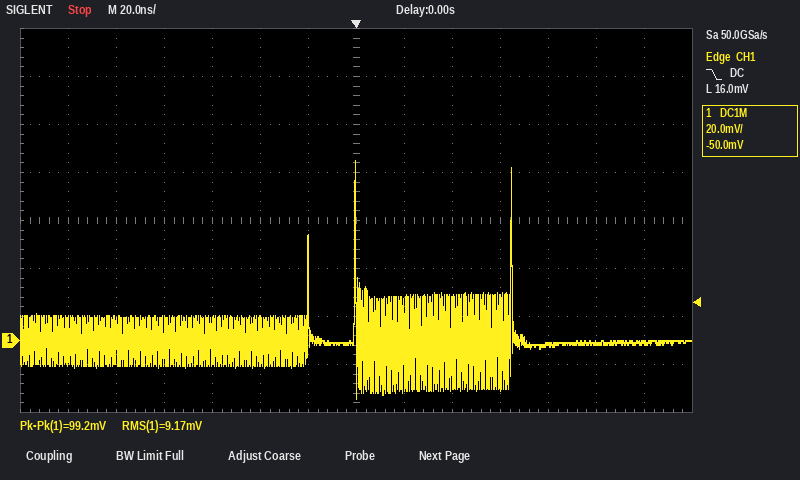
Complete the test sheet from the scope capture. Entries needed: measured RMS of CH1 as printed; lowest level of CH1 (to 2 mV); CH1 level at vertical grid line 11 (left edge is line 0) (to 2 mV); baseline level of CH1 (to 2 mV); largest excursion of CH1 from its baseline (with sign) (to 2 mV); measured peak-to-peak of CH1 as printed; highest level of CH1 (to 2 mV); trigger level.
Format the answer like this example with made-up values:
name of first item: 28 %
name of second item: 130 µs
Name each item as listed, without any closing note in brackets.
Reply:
measured RMS of CH1 as printed: 9.17 mV
lowest level of CH1: -24 mV
CH1 level at vertical grid line 11 (left edge is line 0): -2 mV
baseline level of CH1: 0 mV
largest excursion of CH1 from its baseline (with sign): +76 mV
measured peak-to-peak of CH1 as printed: 99.2 mV
highest level of CH1: 76 mV
trigger level: 16.0 mV
